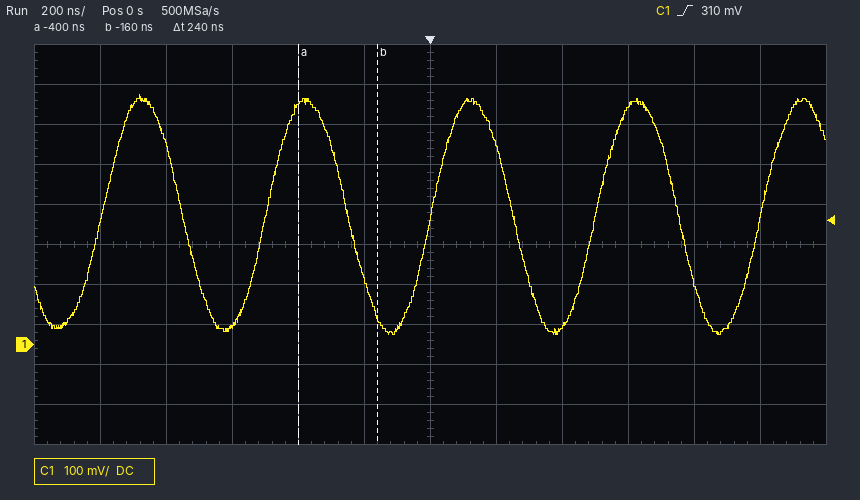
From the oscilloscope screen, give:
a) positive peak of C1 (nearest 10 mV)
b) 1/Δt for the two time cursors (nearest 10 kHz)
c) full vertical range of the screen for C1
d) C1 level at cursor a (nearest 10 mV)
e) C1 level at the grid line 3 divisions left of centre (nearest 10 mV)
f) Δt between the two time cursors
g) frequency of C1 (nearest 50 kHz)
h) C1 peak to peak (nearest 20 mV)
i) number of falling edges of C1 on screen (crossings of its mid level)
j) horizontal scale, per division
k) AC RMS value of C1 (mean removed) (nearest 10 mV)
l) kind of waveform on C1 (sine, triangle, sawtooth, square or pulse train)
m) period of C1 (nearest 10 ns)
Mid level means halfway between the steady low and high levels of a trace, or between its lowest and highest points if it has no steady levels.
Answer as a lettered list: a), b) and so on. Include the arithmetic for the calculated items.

a) 620 mV
b) 1 / 240 ns ≈ 4.17 MHz
c) 1 V
d) 600 mV
e) 50 mV
f) 240 ns
g) 1 / 500 ns ≈ 2.00 MHz
h) 600 mV
i) 4
j) 200 ns
k) 600 mV / (2√2) ≈ 212 mV, so 210 mV to the nearest 10 mV
l) sine
m) 500 ns
